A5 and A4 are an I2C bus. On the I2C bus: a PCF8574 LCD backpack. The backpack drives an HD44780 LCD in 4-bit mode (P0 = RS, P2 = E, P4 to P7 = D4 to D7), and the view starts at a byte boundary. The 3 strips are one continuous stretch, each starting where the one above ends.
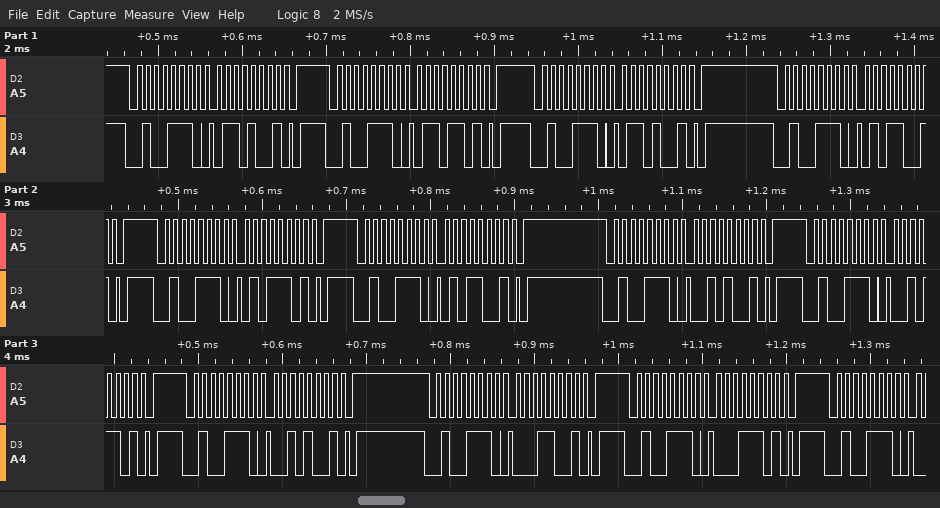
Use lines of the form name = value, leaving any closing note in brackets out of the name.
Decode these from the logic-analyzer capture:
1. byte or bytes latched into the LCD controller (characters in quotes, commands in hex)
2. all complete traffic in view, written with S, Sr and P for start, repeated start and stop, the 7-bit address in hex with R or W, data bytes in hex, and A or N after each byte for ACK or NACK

byte or bytes latched into the LCD controller = 'e'
all complete traffic in view, written with S, Sr and P for start, repeated start and stop, the 7-bit address in hex with R or W, data bytes in hex, and A or N after each byte for ACK or NACK = S 27W A 69 A P S 27W A 6D A P S 27W A 69 A P S 27W A 59 A P S 27W A 5D A P S 27W A 59 A P S 27W A 29 A P S 27W A 2D A P S 27W A 29 A P S 27W A 19 A P S 27W A 1D A P S 27W A
